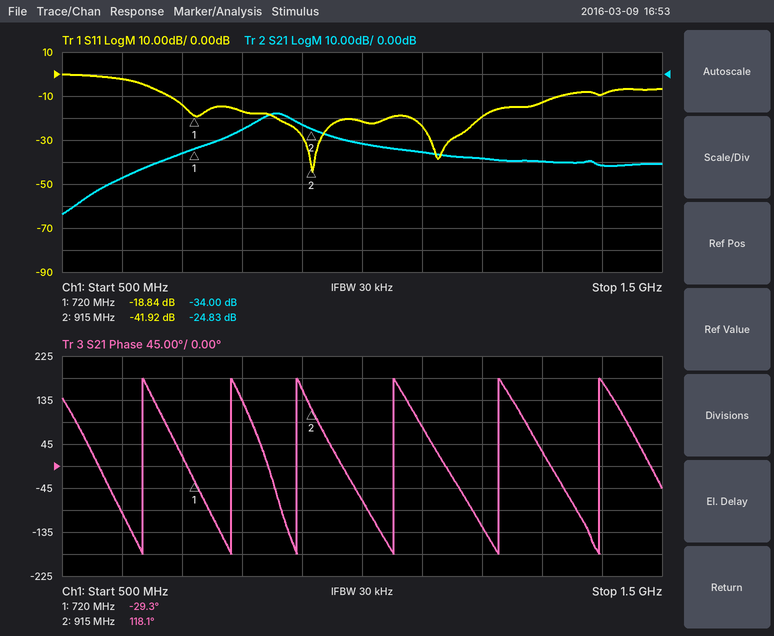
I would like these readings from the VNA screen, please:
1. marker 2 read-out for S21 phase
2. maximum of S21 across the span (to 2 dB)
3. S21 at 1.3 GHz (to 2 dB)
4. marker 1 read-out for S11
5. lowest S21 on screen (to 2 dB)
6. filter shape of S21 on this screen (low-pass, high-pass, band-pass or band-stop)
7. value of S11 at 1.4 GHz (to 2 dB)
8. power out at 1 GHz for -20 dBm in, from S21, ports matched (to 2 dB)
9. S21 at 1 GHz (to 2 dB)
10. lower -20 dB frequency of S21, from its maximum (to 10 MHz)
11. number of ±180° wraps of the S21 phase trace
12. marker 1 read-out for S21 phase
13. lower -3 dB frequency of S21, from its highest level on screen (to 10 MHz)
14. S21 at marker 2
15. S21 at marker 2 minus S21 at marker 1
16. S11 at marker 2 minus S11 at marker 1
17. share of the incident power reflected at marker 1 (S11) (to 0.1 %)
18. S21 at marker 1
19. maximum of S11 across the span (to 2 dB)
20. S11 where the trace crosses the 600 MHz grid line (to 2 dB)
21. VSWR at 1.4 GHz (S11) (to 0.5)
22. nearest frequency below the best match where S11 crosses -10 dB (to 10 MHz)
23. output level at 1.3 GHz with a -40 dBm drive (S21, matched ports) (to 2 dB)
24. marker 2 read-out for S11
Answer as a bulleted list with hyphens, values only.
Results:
- 118.1°
- -18 dB
- -40 dB
- -18.84 dB
- -64 dB
- band-pass
- -10 dB
- -52 dBm
- -32 dB
- 680 MHz
- 6
- -29.3°
- 830 MHz
- -24.83 dB
- 9.17 dB
- -23.08 dB
- 1.3 %
- -34.00 dB
- 0 dB
- -2 dB
- 2.0
- 680 MHz
- -80 dBm
- -41.92 dB
